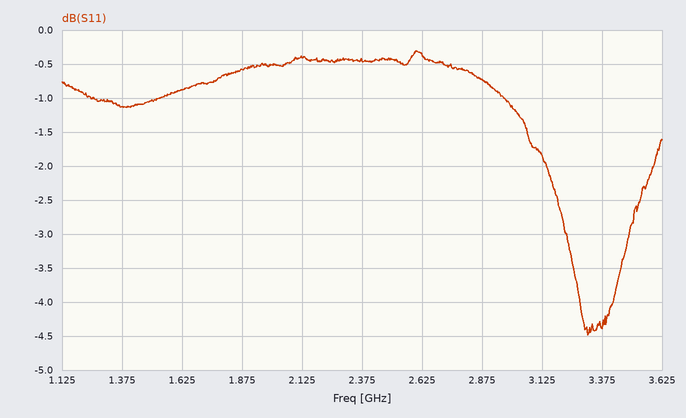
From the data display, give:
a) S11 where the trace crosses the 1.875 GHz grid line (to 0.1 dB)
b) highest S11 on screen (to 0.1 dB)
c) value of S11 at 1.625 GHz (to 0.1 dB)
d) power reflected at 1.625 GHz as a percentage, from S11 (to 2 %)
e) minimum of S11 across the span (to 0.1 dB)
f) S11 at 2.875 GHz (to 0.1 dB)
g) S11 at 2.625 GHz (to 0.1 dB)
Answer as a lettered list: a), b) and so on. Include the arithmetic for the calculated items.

a) -0.6 dB
b) -0.3 dB
c) -0.9 dB
d) 10^(-0.9/10) ≈ 81.3 %, so 82 % to the nearest 2 %
e) -4.5 dB
f) -0.7 dB
g) -0.4 dB
